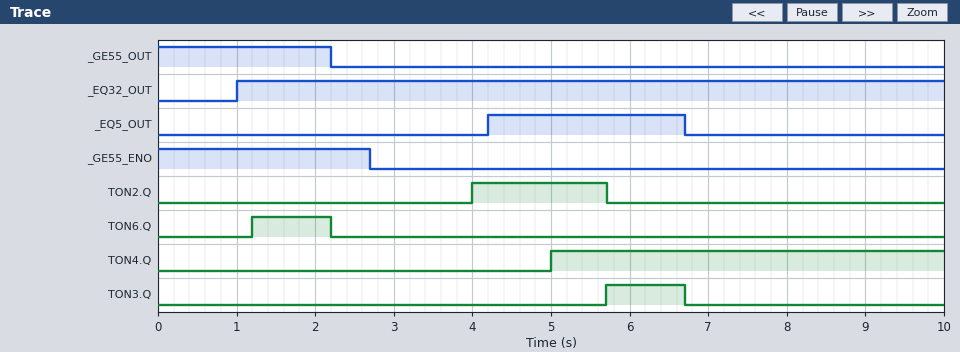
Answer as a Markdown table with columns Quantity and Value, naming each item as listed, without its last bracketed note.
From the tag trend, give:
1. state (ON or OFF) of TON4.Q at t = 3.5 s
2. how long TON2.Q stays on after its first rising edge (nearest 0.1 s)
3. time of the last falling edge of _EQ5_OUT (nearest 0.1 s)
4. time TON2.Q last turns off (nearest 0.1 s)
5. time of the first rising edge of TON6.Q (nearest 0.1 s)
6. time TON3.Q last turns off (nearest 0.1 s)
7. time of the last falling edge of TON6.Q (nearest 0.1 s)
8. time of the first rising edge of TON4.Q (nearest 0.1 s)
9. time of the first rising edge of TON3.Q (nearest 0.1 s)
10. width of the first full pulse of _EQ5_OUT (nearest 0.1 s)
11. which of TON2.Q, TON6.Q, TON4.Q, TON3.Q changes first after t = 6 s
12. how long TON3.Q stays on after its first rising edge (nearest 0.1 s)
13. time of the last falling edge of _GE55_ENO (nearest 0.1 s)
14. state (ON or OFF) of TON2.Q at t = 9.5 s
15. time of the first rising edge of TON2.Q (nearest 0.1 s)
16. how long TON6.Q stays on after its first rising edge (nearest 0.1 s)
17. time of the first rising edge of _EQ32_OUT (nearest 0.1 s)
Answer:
| Quantity | Value |
|---|---|
| state (ON or OFF) of TON4.Q at t = 3.5 s | OFF |
| how long TON2.Q stays on after its first rising edge | 1.7 s |
| time of the last falling edge of _EQ5_OUT | 6.7 s |
| time TON2.Q last turns off | 5.7 s |
| time of the first rising edge of TON6.Q | 1.2 s |
| time TON3.Q last turns off | 6.7 s |
| time of the last falling edge of TON6.Q | 2.2 s |
| time of the first rising edge of TON4.Q | 5.0 s |
| time of the first rising edge of TON3.Q | 5.7 s |
| width of the first full pulse of _EQ5_OUT | 2.5 s |
| which of TON2.Q, TON6.Q, TON4.Q, TON3.Q changes first after t = 6 s | TON3.Q |
| how long TON3.Q stays on after its first rising edge | 1.0 s |
| time of the last falling edge of _GE55_ENO | 2.7 s |
| state (ON or OFF) of TON2.Q at t = 9.5 s | OFF |
| time of the first rising edge of TON2.Q | 4.0 s |
| how long TON6.Q stays on after its first rising edge | 1.0 s |
| time of the first rising edge of _EQ32_OUT | 1.0 s |
